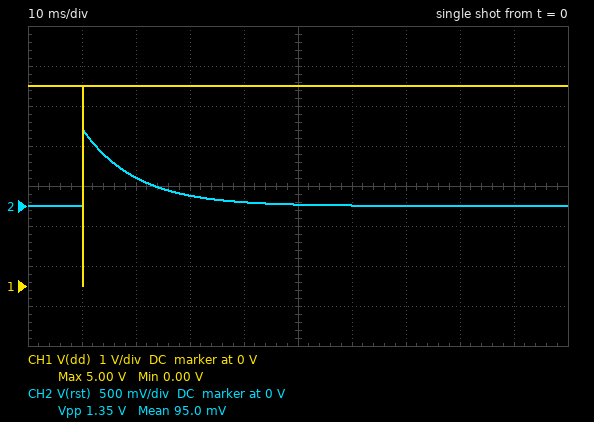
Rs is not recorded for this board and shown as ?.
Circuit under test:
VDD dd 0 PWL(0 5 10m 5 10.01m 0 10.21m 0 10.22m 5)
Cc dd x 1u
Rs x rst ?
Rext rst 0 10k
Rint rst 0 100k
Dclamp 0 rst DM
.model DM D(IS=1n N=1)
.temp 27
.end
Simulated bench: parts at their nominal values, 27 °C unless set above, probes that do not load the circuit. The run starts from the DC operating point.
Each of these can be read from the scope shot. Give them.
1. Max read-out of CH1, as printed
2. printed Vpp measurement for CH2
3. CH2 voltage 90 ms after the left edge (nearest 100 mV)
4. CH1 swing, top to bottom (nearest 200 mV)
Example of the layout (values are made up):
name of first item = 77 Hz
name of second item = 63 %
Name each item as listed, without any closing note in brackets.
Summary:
Max read-out of CH1, as printed = 5.00 V
printed Vpp measurement for CH2 = 1.35 V
CH2 voltage 90 ms after the left edge = 0 V
CH1 swing, top to bottom = 5.0 V
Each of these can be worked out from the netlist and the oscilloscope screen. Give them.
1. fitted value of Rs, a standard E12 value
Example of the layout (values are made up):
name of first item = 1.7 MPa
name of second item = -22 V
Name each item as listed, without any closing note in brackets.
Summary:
fitted value of Rs, a standard E12 value = 820 Ω
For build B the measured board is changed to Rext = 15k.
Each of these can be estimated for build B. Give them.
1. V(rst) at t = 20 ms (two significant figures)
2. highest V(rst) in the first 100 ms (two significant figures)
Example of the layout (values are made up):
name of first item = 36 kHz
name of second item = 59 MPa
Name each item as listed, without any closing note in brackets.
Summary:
V(rst) at t = 20 ms = 480 mV
highest V(rst) in the first 100 ms = 970 mV
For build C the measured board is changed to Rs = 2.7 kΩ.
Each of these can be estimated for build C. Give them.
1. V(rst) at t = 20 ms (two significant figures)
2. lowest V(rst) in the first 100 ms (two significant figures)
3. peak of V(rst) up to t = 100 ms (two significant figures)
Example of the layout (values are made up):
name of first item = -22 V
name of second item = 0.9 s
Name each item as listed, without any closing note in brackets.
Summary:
V(rst) at t = 20 ms = 120 mV
lowest V(rst) in the first 100 ms = -370 mV
peak of V(rst) up to t = 100 ms = 270 mV
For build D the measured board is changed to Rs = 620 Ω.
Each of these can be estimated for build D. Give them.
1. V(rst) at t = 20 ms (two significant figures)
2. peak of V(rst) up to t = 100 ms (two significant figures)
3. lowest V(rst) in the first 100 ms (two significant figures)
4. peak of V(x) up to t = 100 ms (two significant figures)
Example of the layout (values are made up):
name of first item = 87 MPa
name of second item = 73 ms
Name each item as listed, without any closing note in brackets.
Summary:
V(rst) at t = 20 ms = 450 mV
peak of V(rst) up to t = 100 ms = 1.2 V
lowest V(rst) in the first 100 ms = -410 mV
peak of V(x) up to t = 100 ms = 1.3 V
